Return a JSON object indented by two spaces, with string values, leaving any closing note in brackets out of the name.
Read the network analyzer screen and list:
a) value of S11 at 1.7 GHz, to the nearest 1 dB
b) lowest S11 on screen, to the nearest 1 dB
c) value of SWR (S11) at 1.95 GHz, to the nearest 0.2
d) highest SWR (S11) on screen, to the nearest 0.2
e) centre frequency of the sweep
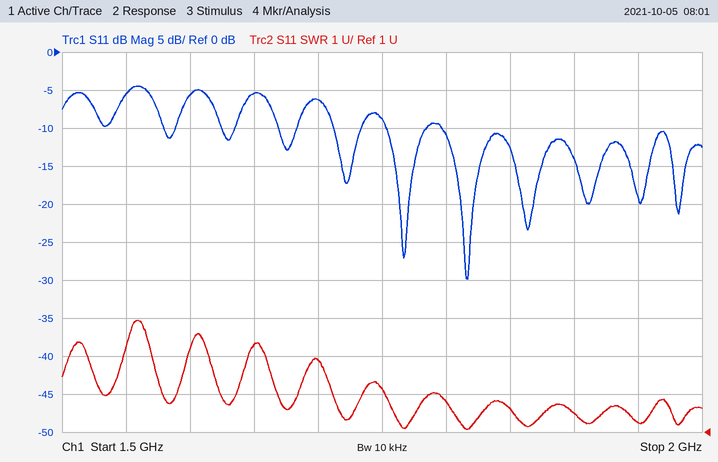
{
  "value of S11 at 1.7 GHz, to the nearest 1 dB": "-6 dB",
  "lowest S11 on screen, to the nearest 1 dB": "-30 dB",
  "value of SWR (S11) at 1.95 GHz, to the nearest 0.2": "1.2",
  "highest SWR (S11) on screen, to the nearest 0.2": "4.0",
  "centre frequency of the sweep": "1.75 GHz"
}
